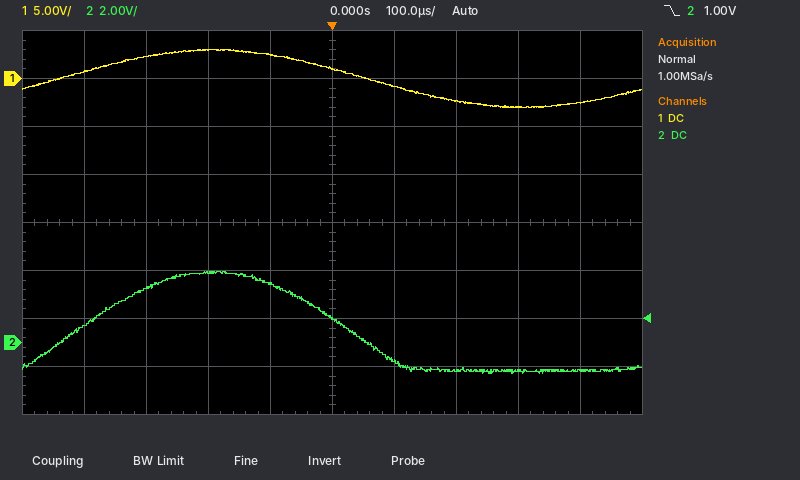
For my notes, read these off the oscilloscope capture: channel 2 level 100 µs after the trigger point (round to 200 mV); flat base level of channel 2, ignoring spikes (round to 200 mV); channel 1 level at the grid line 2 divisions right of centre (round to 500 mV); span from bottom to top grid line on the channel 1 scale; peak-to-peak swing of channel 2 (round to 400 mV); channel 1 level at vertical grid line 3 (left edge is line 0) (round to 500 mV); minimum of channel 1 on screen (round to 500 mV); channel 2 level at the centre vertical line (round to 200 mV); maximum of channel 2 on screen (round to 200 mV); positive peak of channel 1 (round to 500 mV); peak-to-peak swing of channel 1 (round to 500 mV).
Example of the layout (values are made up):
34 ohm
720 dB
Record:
-800 mV
-1.2 V
-2.5 V
40 V
4.4 V
3.0 V
-3.0 V
1.0 V
3.0 V
3.0 V
6.0 V
